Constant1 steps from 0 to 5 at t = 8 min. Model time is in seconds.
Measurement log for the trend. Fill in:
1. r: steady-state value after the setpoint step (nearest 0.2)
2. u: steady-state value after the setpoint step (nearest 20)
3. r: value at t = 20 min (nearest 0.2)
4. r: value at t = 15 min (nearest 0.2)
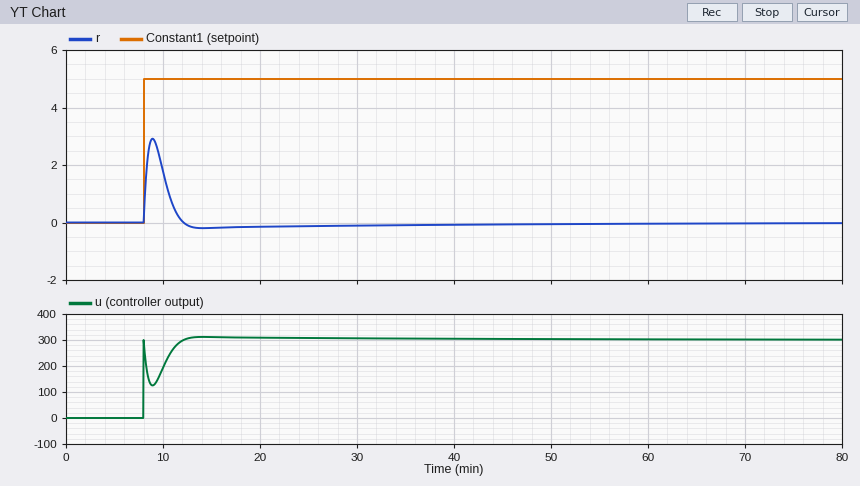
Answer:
0.0
300
-0.2
-0.2
